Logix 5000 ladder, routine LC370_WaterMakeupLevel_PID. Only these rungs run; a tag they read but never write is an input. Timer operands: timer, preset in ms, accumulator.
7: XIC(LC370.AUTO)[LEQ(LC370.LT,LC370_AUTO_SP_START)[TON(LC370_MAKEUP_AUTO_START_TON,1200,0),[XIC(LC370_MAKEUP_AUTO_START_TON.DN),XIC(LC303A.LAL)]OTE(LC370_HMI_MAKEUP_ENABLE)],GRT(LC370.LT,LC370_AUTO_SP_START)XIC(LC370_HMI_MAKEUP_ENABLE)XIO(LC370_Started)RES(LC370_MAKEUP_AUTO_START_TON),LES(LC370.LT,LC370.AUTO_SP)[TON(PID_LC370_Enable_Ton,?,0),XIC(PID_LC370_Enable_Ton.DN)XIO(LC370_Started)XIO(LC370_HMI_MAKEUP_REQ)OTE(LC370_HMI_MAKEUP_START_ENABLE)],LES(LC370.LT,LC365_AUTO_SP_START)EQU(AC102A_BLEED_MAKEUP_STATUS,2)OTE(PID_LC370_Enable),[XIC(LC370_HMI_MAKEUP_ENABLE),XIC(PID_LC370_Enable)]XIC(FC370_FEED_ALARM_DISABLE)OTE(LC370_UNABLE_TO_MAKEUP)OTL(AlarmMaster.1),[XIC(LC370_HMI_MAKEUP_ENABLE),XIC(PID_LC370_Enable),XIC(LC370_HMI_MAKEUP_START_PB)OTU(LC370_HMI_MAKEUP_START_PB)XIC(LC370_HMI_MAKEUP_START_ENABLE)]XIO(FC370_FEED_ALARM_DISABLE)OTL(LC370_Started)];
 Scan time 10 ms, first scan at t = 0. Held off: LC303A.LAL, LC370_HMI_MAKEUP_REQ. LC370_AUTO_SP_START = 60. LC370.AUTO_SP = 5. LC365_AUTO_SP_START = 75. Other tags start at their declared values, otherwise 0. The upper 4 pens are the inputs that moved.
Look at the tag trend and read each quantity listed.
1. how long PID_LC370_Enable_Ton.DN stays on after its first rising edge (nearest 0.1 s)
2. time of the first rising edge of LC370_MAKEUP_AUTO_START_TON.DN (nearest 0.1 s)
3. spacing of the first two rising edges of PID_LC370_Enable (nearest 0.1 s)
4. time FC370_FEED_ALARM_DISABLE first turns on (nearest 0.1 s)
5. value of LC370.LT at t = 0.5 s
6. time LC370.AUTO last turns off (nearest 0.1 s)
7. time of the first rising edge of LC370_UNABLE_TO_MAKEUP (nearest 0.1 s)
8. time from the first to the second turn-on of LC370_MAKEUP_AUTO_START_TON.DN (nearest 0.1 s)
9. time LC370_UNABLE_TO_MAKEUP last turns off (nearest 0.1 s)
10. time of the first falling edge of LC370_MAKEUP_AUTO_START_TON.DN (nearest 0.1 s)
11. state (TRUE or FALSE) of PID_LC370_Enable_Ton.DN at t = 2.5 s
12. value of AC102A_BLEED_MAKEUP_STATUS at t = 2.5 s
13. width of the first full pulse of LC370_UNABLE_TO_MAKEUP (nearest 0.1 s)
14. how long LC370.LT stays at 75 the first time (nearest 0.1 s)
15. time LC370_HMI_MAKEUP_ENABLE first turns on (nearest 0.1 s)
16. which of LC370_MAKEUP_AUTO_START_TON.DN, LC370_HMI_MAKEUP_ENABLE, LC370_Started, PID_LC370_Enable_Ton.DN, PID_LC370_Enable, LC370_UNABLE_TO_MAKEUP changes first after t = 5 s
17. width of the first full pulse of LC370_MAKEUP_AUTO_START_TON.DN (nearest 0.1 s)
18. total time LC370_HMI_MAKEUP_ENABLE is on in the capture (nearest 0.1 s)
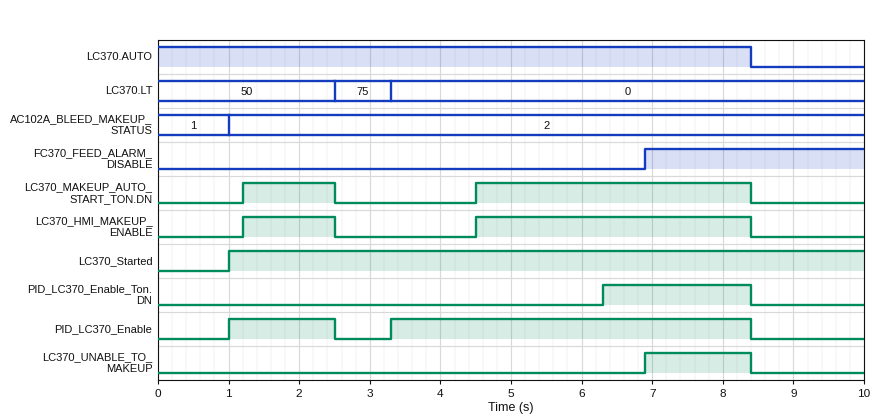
2.1 s
1.2 s
2.3 s
6.9 s
50
8.4 s
6.9 s
3.3 s
8.4 s
2.5 s
FALSE
2
1.5 s
0.8 s
1.2 s
PID_LC370_Enable_Ton.DN
1.3 s
5.2 s
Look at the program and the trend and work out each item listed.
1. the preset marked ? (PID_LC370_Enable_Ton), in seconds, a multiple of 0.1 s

3.0 s
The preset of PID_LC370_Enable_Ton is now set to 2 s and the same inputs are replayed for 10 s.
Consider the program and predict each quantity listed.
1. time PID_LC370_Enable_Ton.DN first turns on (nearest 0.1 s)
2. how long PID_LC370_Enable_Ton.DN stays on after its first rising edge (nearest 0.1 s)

5.3 s
3.1 s
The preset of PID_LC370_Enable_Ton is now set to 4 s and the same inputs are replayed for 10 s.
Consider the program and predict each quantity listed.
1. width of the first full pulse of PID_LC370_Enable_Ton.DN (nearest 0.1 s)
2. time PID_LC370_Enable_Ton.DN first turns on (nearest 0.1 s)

1.1 s
7.3 s
